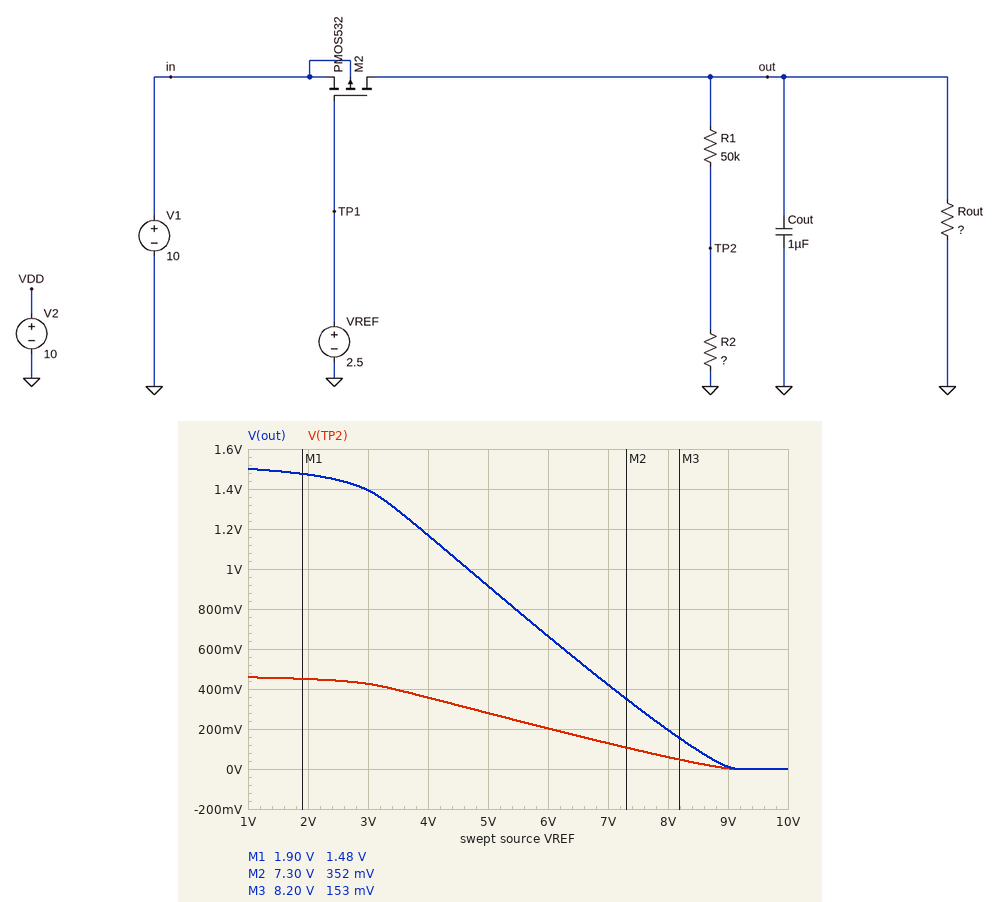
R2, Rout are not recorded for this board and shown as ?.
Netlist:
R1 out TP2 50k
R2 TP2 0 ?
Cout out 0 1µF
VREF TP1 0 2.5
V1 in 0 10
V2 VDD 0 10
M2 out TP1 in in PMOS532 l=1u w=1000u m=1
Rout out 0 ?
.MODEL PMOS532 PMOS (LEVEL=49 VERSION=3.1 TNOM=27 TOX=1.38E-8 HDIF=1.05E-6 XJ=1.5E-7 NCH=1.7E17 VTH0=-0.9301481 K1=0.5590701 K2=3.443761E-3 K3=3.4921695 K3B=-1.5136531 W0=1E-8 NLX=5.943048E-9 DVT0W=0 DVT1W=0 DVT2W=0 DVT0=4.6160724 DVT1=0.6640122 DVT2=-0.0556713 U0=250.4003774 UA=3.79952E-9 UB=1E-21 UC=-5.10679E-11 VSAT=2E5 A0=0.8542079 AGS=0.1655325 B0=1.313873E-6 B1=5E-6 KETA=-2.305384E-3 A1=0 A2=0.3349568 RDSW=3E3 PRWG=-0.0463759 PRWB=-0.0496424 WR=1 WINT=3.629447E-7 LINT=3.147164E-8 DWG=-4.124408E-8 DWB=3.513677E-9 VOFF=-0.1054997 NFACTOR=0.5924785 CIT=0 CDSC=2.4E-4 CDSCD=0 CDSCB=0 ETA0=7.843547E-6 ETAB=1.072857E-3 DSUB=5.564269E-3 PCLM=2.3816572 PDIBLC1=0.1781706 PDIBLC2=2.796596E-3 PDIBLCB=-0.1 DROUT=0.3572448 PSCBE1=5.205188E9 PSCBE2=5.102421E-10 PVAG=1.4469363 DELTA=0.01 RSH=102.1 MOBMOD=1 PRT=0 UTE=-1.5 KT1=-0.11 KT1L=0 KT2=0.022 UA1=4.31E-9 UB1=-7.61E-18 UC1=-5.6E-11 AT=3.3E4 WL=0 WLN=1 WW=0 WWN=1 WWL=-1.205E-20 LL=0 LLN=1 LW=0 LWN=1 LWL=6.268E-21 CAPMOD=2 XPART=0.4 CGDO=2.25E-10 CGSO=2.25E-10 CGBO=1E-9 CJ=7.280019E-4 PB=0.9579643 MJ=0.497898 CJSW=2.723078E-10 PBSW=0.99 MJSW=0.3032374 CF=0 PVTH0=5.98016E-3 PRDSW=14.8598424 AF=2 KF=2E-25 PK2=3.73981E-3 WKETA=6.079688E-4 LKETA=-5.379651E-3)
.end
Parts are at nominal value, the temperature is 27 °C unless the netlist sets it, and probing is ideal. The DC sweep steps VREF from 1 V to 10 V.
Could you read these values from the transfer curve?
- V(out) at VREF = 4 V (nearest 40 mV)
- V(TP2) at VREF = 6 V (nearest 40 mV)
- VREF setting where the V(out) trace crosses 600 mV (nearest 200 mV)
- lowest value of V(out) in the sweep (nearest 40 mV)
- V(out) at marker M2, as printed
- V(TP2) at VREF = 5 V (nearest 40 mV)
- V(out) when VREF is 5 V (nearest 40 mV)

1.16 V
200 mV
6.2 V
0 V
352 mV
280 mV
920 mV
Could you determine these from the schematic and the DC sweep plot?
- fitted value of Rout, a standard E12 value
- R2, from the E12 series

39 Ω
22 kΩ
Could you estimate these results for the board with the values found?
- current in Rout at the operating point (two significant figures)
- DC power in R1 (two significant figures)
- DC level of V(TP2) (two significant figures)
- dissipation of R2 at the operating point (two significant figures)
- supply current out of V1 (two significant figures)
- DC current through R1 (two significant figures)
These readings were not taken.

37 mA
20 µW
440 mV
8.9 µW
37 mA
20 µA
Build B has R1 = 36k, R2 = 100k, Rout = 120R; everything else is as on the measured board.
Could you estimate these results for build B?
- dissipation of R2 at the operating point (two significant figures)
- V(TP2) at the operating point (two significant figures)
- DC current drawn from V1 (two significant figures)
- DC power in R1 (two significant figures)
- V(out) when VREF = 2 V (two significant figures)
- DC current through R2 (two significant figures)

67 µW
2.6 V
29 mA
24 µW
3.5 V
26 µA
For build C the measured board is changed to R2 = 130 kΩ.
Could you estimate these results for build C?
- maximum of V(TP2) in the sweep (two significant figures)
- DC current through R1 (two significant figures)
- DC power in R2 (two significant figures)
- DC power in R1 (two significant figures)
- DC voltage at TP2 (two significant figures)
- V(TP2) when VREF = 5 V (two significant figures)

1.1 V
8.0 µA
8.4 µW
3.2 µW
1.0 V
660 mV
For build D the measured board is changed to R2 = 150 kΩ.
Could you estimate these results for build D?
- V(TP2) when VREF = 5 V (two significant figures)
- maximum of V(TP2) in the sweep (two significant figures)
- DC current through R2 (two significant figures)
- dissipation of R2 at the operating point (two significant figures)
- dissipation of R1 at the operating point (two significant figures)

690 mV
1.1 V
7.2 µA
7.8 µW
2.6 µW
